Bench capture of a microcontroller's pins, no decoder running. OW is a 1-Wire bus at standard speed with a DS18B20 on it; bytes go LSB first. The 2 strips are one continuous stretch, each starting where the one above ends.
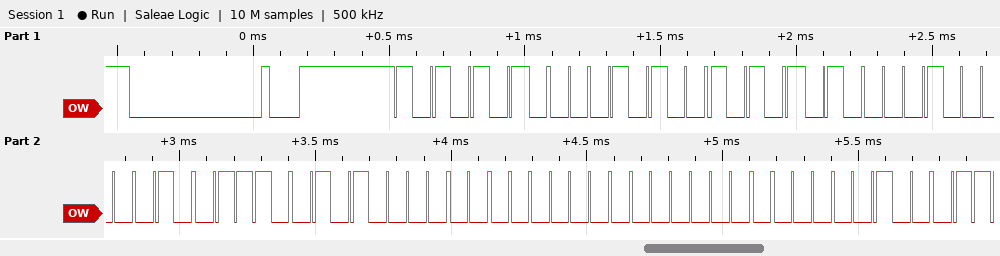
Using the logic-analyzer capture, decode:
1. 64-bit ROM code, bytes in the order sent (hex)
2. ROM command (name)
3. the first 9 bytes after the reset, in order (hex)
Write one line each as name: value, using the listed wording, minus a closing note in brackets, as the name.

64-bit ROM code, bytes in the order sent: 28 55 08 72 0A 00 00 20
ROM command: Match ROM
the first 9 bytes after the reset, in order: 55 28 55 08 72 0A 00 00 20
